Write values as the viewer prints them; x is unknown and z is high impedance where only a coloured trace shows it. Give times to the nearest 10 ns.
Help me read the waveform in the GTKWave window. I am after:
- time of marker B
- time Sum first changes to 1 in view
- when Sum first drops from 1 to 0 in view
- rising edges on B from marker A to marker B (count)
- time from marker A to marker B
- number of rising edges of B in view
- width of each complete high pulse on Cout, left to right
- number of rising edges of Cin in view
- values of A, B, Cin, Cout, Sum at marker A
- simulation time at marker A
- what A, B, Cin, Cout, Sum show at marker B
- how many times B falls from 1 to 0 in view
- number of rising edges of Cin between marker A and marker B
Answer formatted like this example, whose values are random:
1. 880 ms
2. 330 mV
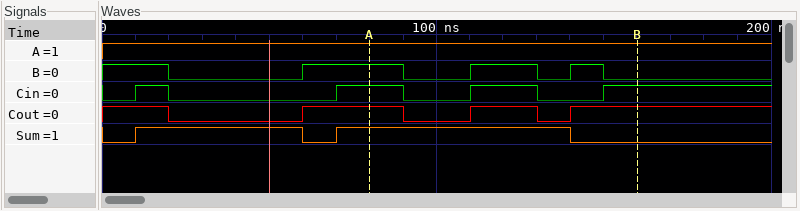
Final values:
1. 160 ns
2. 10 ns
3. 60 ns
4. 2
5. 80 ns
6. 3
7. 30 ns, 20 ns
8. 4
9. A=1, B=1, Cin=1, Cout=1, Sum=1
10. 80 ns
11. A=1, B=0, Cin=1, Cout=1, Sum=0
12. 4
13. 2
